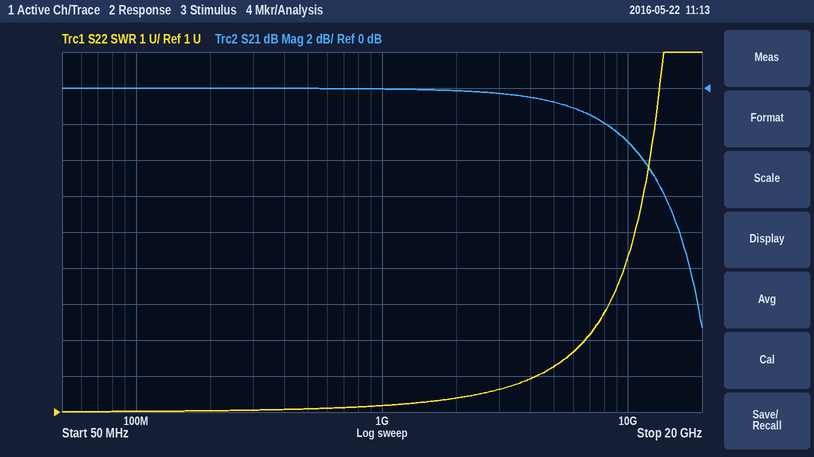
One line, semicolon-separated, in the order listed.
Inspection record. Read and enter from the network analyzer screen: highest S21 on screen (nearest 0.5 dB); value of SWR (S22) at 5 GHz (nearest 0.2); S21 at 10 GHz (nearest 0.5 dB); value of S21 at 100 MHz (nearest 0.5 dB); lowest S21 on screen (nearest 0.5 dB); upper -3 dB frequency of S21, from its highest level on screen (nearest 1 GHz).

0.0 dB; 2.2; -3.0 dB; 0.0 dB; -13.5 dB; 10 GHz
